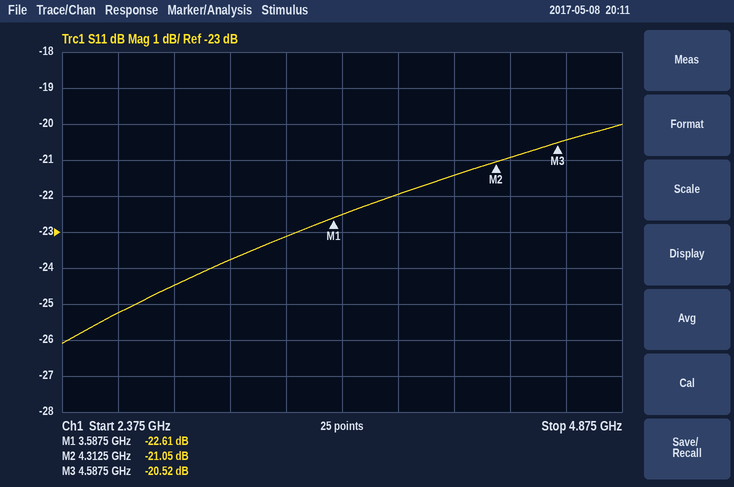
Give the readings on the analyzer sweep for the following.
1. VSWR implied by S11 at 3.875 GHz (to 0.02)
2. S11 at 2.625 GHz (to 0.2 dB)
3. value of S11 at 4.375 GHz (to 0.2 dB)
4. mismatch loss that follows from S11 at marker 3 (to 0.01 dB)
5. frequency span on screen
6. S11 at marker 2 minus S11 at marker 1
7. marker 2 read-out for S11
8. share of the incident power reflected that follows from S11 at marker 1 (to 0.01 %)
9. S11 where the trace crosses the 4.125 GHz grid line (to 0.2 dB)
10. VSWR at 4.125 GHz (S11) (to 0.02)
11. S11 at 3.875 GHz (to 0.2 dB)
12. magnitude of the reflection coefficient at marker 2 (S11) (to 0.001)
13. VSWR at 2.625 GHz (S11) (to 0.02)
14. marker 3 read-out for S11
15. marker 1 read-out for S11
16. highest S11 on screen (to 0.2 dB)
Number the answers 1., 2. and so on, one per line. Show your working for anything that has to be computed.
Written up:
1. |Γ| = 10^(-22/20) = 0.0794; VSWR = (1 + 0.0794)/(1 − 0.0794) ≈ 1.17, so 1.18 to the nearest 0.02
2. -25.2 dB
3. -21.0 dB
4. −10 log10(1 − 10^(-20.52/10)) ≈ 0.04 dB
5. 2.5 GHz
6. -21.05 − (-22.61) = 1.56 dB
7. -21.05 dB
8. 10^(-22.61/10) ≈ 0.55 %
9. -21.4 dB
10. |Γ| = 10^(-21.4/20) = 0.0851; VSWR = (1 + 0.0851)/(1 − 0.0851) ≈ 1.19, so 1.18 to the nearest 0.02
11. -22.0 dB
12. 10^(-21.05/20) ≈ 0.089
13. |Γ| = 10^(-25.2/20) = 0.0550; VSWR = (1 + 0.0550)/(1 − 0.0550) ≈ 1.12
14. -20.52 dB
15. -22.61 dB
16. -20.0 dB
